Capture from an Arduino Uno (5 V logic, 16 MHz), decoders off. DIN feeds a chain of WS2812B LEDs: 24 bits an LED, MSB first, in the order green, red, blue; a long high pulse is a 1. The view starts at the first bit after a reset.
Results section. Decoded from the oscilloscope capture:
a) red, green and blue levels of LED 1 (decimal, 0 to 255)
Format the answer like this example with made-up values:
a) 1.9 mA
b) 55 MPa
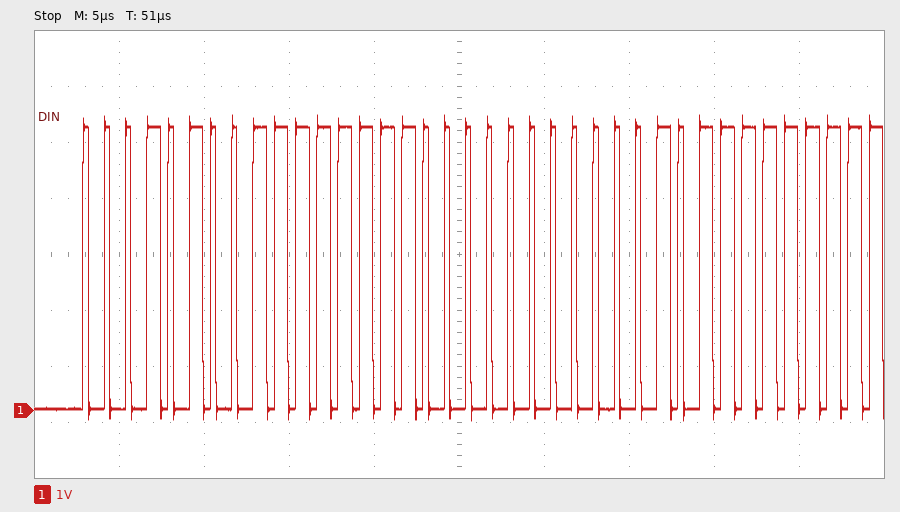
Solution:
a) 255, 20, 0
